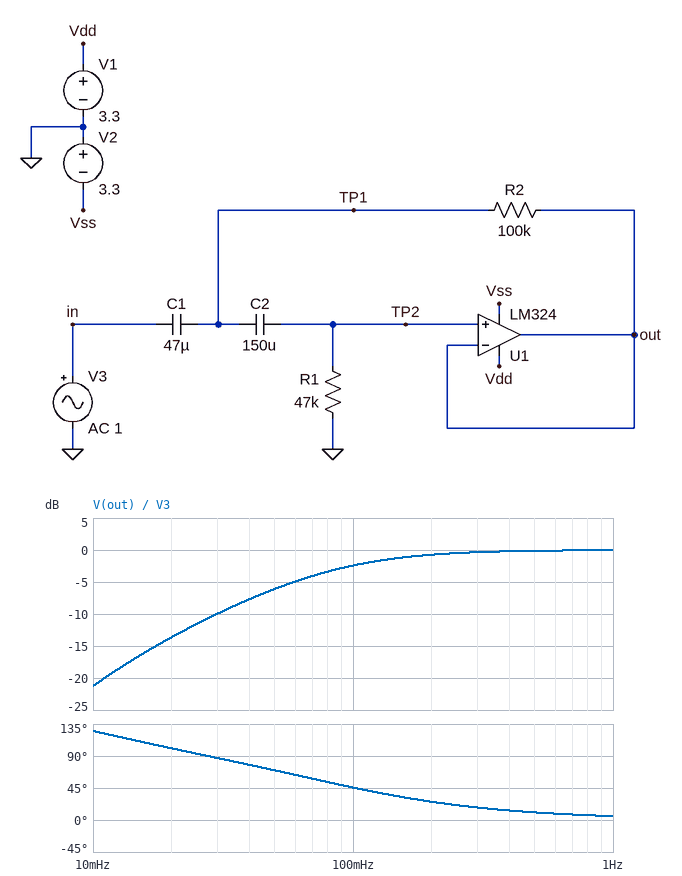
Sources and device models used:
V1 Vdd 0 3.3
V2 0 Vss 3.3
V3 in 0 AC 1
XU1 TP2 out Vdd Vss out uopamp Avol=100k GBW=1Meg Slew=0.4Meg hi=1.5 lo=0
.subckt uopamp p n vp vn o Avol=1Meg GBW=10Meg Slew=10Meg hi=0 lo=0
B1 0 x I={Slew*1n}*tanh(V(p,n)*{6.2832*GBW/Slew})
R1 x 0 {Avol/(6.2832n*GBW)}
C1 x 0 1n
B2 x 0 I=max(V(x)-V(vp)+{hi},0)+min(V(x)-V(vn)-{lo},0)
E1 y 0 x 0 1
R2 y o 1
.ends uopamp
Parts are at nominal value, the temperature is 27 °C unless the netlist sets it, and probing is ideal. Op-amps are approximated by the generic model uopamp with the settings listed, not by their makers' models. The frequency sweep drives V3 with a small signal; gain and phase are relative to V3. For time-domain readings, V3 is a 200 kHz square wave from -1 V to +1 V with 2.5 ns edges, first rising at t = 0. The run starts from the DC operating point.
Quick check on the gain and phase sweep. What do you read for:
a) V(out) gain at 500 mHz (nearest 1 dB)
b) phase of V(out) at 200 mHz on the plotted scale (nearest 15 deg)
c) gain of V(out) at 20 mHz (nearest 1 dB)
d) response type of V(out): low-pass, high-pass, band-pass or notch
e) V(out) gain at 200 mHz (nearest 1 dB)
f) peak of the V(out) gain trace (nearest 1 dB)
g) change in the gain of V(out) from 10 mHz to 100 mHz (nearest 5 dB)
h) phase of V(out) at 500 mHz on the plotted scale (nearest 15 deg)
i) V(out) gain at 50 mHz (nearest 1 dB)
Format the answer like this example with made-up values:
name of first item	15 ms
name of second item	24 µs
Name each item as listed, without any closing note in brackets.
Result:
V(out) gain at 500 mHz	0 dB
phase of V(out) at 200 mHz on the plotted scale	30 deg
gain of V(out) at 20 mHz	-14 dB
response type of V(out): low-pass, high-pass, band-pass or notch	high-pass
V(out) gain at 200 mHz	-1 dB
peak of the V(out) gain trace	0 dB
change in the gain of V(out) from 10 mHz to 100 mHz	20 dB
phase of V(out) at 500 mHz on the plotted scale	15 deg
V(out) gain at 50 mHz	-6 dB
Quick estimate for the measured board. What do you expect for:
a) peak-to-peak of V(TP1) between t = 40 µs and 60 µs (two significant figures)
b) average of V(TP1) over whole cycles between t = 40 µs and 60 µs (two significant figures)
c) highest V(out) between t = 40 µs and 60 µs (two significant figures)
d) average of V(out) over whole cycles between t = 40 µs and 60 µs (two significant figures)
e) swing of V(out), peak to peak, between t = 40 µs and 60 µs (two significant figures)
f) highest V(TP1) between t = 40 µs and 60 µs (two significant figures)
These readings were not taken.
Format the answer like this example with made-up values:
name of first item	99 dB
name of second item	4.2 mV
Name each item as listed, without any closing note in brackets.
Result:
peak-to-peak of V(TP1) between t = 40 µs and 60 µs	2.0 V
average of V(TP1) over whole cycles between t = 40 µs and 60 µs	1.0 V
highest V(out) between t = 40 µs and 60 µs	1.1 V
average of V(out) over whole cycles between t = 40 µs and 60 µs	600 mV
swing of V(out), peak to peak, between t = 40 µs and 60 µs	1.0 V
highest V(TP1) between t = 40 µs and 60 µs	2.0 V
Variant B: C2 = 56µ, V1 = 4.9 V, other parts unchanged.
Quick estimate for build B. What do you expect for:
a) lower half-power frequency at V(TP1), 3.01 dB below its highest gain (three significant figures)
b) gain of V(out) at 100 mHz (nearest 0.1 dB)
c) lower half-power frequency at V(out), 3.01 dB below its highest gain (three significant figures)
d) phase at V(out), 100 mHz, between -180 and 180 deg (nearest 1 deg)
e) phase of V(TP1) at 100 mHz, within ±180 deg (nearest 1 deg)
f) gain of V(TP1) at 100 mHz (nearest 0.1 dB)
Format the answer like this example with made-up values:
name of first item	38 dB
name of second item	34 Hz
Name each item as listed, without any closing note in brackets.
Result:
lower half-power frequency at V(TP1), 3.01 dB below its highest gain	82.3 mHz
gain of V(out) at 100 mHz	-3.8 dB
lower half-power frequency at V(out), 3.01 dB below its highest gain	117 mHz
phase at V(out), 100 mHz, between -180 and 180 deg	59 deg
phase of V(TP1) at 100 mHz, within ±180 deg	28 deg
gain of V(TP1) at 100 mHz	-2.4 dB
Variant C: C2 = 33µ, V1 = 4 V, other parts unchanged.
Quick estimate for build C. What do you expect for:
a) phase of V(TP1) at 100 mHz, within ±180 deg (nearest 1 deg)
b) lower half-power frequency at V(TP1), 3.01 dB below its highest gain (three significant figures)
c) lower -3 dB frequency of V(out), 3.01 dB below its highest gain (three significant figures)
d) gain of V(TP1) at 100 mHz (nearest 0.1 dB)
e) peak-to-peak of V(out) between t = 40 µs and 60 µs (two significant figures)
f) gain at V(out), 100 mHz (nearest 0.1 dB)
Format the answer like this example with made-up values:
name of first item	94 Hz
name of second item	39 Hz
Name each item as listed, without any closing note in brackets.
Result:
phase of V(TP1) at 100 mHz, within ±180 deg	24 deg
lower half-power frequency at V(TP1), 3.01 dB below its highest gain	70.3 mHz
lower -3 dB frequency of V(out), 3.01 dB below its highest gain	155 mHz
gain of V(TP1) at 100 mHz	-2.3 dB
peak-to-peak of V(out) between t = 40 µs and 60 µs	1.0 V
gain at V(out), 100 mHz	-5.4 dB
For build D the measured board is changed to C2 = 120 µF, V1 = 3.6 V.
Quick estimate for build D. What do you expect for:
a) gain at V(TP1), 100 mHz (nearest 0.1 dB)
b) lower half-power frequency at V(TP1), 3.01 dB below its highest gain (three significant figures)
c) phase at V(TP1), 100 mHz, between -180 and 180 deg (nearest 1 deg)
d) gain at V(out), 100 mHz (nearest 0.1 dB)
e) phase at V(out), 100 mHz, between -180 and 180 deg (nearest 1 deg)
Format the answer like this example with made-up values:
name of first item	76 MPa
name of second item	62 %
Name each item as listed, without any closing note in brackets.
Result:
gain at V(TP1), 100 mHz	-2.3 dB
lower half-power frequency at V(TP1), 3.01 dB below its highest gain	81.8 mHz
phase at V(TP1), 100 mHz, between -180 and 180 deg	32 deg
gain at V(out), 100 mHz	-2.6 dB
phase at V(out), 100 mHz, between -180 and 180 deg	48 deg
